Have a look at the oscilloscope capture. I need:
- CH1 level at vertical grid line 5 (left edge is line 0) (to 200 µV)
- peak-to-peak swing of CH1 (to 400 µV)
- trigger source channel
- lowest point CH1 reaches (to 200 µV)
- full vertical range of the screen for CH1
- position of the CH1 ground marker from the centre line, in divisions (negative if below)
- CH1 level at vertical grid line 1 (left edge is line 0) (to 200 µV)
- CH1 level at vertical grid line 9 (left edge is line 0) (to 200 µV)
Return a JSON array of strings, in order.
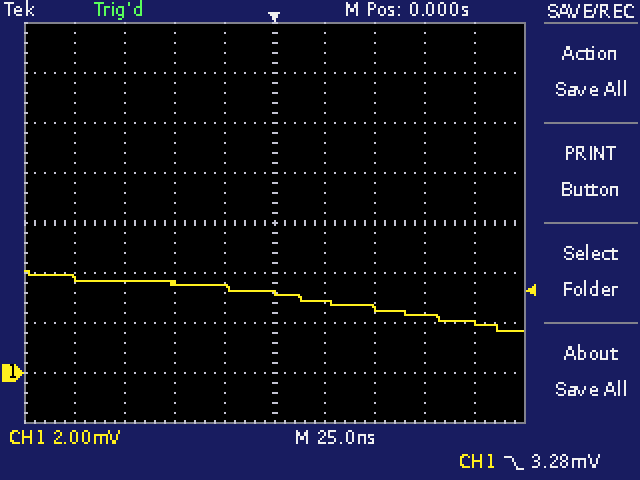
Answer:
["3.2 mV", "2.4 mV", "CH1", "1.6 mV", "16 mV", "-3.0 div", "3.8 mV", "2.0 mV"]
